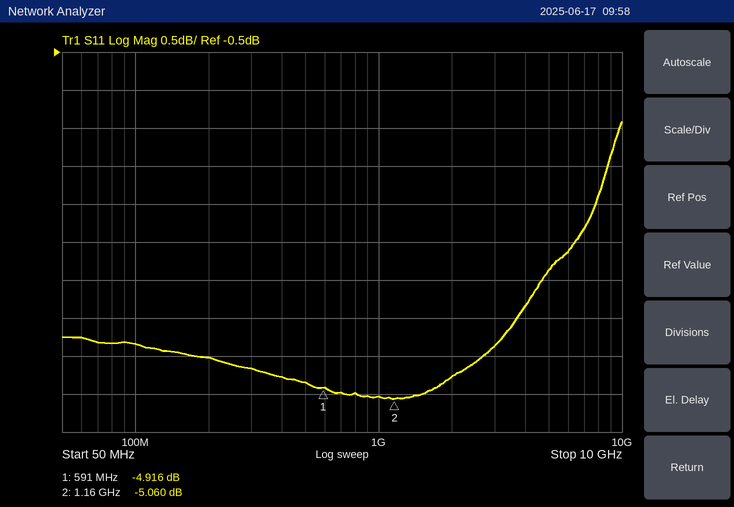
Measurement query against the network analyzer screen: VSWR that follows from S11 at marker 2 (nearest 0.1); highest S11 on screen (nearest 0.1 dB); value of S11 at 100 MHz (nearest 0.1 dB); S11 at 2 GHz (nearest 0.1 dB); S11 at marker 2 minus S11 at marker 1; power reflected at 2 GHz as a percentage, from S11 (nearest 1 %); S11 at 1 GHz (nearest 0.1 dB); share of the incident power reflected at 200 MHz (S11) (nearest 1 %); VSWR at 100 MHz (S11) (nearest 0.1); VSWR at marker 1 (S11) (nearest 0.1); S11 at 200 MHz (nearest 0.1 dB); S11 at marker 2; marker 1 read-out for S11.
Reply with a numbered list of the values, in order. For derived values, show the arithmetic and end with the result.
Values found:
1. (1 + 0.5585)/(1 − 0.5585) ≈ 3.5
2. -1.4 dB
3. -4.3 dB
4. -4.8 dB
5. -5.06 − (-4.916) = -0.144 dB
6. 10^(-4.8/10) ≈ 33 %
7. -5.0 dB
8. 10^(-4.5/10) ≈ 35 %
9. |Γ| = 10^(-4.3/20) = 0.6095; VSWR = (1 + 0.6095)/(1 − 0.6095) ≈ 4.1
10. (1 + 0.5678)/(1 − 0.5678) ≈ 3.6
11. -4.5 dB
12. -5.060 dB
13. -4.916 dB
